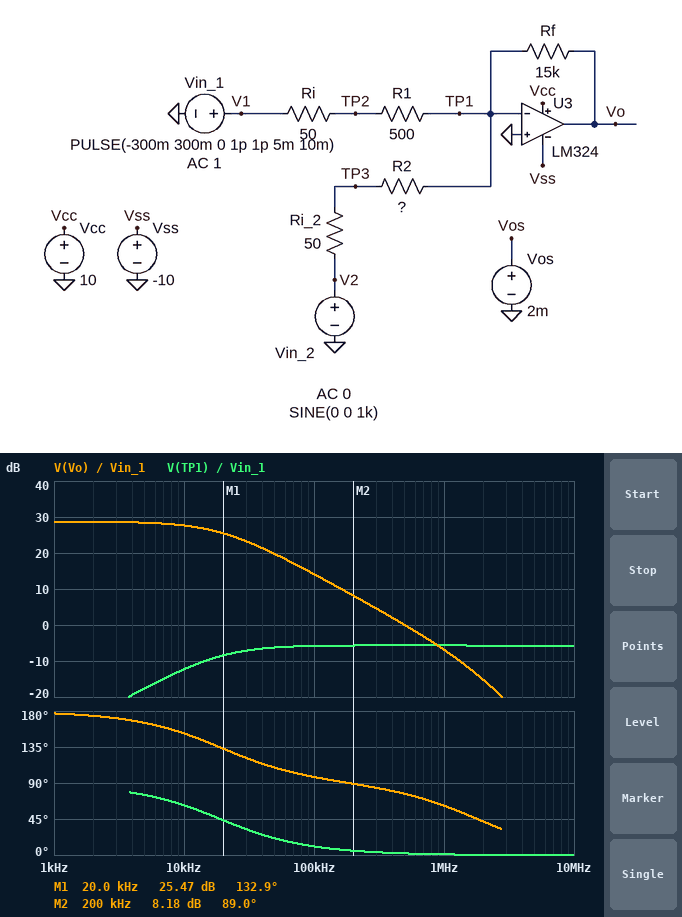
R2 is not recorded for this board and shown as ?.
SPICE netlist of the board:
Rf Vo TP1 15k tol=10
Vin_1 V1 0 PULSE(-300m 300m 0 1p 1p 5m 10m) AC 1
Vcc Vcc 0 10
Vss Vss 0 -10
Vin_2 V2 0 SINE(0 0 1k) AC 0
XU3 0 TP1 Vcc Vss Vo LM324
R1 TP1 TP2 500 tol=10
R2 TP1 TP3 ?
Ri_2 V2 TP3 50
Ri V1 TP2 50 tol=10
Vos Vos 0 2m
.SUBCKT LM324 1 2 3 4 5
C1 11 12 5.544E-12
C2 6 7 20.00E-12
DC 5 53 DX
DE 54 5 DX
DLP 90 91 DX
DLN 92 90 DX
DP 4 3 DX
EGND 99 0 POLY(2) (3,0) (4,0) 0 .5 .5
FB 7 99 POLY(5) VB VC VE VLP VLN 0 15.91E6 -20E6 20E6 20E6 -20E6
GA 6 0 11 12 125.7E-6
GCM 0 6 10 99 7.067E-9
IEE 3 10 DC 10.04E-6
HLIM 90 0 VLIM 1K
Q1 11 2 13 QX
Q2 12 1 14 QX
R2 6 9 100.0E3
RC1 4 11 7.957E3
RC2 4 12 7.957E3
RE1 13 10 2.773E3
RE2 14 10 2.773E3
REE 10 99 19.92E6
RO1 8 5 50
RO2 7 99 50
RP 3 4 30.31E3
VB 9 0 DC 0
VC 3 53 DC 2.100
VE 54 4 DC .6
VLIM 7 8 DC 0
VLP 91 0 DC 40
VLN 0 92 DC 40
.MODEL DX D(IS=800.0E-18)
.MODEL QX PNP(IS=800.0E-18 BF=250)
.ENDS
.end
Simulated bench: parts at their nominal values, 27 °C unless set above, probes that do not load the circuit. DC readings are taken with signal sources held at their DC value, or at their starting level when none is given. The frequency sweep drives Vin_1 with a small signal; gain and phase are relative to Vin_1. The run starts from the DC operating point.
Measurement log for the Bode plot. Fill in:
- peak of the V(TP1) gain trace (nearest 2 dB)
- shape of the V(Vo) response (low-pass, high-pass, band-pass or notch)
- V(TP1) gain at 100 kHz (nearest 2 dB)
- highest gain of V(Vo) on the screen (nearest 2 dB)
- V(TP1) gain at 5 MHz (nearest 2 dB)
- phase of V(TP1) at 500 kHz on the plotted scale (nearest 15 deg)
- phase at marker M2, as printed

-6 dB
low-pass
-6 dB
28 dB
-6 dB
0 deg
89.0 deg
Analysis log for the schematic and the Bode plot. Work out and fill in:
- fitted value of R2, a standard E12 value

560 Ω
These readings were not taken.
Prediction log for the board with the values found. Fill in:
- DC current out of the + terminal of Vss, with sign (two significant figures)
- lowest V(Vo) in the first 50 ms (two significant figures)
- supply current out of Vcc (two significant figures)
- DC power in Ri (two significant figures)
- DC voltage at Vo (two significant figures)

-670 µA
-8.2 V
670 µA
15 µW
8.2 V
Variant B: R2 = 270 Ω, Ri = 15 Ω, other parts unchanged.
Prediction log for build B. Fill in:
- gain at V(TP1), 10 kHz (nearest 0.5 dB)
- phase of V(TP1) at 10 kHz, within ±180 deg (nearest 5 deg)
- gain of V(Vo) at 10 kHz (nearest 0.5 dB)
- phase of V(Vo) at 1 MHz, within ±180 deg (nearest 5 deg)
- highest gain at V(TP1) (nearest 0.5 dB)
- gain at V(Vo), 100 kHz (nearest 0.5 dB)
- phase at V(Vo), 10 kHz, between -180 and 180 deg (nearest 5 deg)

-9.0 dB
0 deg
7.0 dB
65 deg
-8.5 dB
1.0 dB
170 deg
